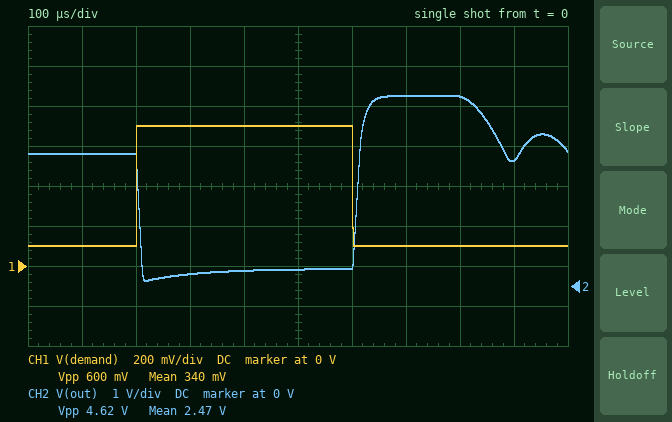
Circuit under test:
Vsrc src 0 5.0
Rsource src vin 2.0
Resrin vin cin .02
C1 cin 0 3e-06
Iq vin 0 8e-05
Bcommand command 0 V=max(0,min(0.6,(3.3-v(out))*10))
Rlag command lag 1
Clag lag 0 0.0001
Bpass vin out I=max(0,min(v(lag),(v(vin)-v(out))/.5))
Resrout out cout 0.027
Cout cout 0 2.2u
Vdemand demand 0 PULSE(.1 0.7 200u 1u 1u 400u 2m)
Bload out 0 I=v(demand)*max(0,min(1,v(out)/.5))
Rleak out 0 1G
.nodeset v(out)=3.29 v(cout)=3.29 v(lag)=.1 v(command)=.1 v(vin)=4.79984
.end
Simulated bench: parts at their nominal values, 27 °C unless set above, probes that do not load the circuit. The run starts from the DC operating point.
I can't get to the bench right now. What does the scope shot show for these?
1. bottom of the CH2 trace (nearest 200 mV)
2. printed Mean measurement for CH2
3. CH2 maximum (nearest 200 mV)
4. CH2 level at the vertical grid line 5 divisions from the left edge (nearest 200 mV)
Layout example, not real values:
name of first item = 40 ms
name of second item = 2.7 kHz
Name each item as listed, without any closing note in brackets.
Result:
bottom of the CH2 trace = 200 mV
printed Mean measurement for CH2 = 2.47 V
CH2 maximum = 4.8 V
CH2 level at the vertical grid line 5 divisions from the left edge = 400 mV
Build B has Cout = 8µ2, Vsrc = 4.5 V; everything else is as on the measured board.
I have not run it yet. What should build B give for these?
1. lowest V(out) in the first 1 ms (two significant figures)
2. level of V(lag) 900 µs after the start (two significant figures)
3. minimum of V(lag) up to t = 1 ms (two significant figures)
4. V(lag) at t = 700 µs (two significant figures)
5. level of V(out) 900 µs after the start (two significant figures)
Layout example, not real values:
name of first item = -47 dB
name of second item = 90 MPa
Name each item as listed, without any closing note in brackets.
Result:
lowest V(out) in the first 1 ms = 240 mV
level of V(lag) 900 µs after the start = 49 mV
minimum of V(lag) up to t = 1 ms = 21 mV
V(lag) at t = 700 µs = 360 mV
level of V(out) 900 µs after the start = 4.0 V
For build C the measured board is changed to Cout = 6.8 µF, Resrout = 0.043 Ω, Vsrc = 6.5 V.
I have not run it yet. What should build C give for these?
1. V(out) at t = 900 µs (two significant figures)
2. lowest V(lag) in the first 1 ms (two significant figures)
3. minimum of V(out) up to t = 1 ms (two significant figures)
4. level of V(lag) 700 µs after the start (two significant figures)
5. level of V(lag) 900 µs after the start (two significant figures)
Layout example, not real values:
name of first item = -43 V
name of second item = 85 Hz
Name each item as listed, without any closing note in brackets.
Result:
V(out) at t = 900 µs = 5.9 V
lowest V(lag) in the first 1 ms = 16 mV
minimum of V(out) up to t = 1 ms = 220 mV
level of V(lag) 700 µs after the start = 330 mV
level of V(lag) 900 µs after the start = 44 mV
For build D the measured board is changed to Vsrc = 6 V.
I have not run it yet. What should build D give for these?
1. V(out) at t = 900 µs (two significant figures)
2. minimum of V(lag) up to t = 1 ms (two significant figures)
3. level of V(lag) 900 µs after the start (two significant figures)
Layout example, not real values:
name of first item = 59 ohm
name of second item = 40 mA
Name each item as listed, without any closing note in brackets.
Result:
V(out) at t = 900 µs = 3.8 V
minimum of V(lag) up to t = 1 ms = 29 mV
level of V(lag) 900 µs after the start = 34 mV
